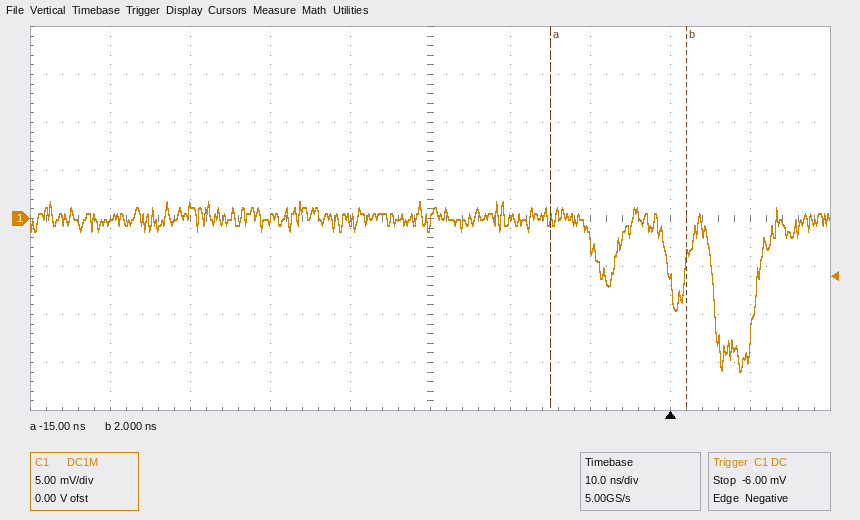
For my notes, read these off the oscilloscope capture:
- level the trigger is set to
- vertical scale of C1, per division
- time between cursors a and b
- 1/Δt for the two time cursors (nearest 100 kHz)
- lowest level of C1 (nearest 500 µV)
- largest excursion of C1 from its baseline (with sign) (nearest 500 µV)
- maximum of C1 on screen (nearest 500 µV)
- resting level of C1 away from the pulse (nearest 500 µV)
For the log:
-6.00 mV
5 mV
17 ns
58.8 MHz
-16.0 mV
-16.0 mV
2.0 mV
0.0 mV
